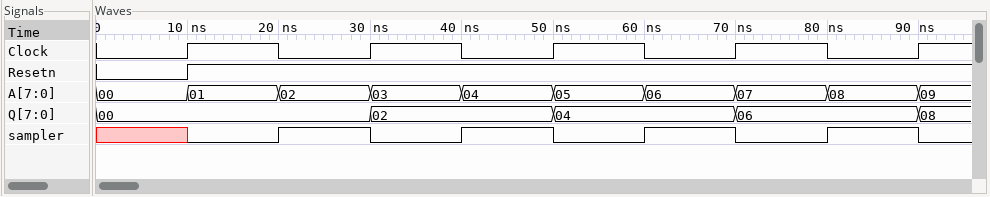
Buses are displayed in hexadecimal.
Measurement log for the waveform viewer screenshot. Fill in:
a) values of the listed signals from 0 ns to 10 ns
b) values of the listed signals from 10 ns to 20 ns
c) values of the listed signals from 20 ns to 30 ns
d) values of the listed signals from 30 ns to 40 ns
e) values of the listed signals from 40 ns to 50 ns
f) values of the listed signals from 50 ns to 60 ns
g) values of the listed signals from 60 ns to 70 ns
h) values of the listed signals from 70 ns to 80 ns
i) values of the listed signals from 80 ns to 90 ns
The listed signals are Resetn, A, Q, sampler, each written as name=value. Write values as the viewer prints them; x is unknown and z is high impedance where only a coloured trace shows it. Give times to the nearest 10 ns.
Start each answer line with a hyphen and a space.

- Resetn=0, A=00, Q=00, sampler=x
- Resetn=1, A=01, Q=00, sampler=0
- Resetn=1, A=02, Q=00, sampler=1
- Resetn=1, A=03, Q=02, sampler=0
- Resetn=1, A=04, Q=02, sampler=1
- Resetn=1, A=05, Q=04, sampler=0
- Resetn=1, A=06, Q=04, sampler=1
- Resetn=1, A=07, Q=06, sampler=0
- Resetn=1, A=08, Q=06, sampler=1
